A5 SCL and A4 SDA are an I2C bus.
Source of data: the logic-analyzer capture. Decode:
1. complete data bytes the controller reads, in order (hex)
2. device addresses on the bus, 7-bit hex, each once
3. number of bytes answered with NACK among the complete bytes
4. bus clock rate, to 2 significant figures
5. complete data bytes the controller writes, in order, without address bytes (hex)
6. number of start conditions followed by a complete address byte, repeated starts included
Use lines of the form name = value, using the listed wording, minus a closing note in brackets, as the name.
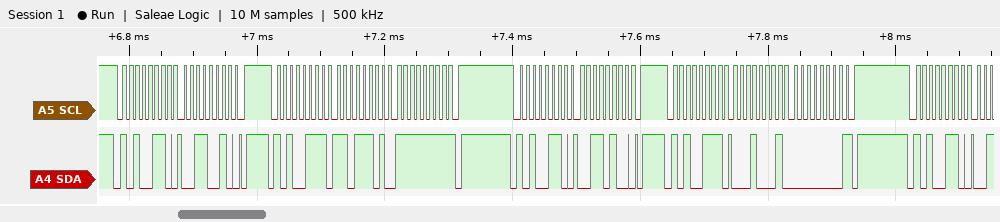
complete data bytes the controller reads, in order = DD FF 11 00
device addresses on the bus, 7-bit hex, each once = 0x53
number of bytes answered with NACK among the complete bytes = 2
bus clock rate, to 2 significant figures = 100 kHz
complete data bytes the controller writes, in order, without address bytes = 32 34
number of start conditions followed by a complete address byte, repeated starts included = 5
